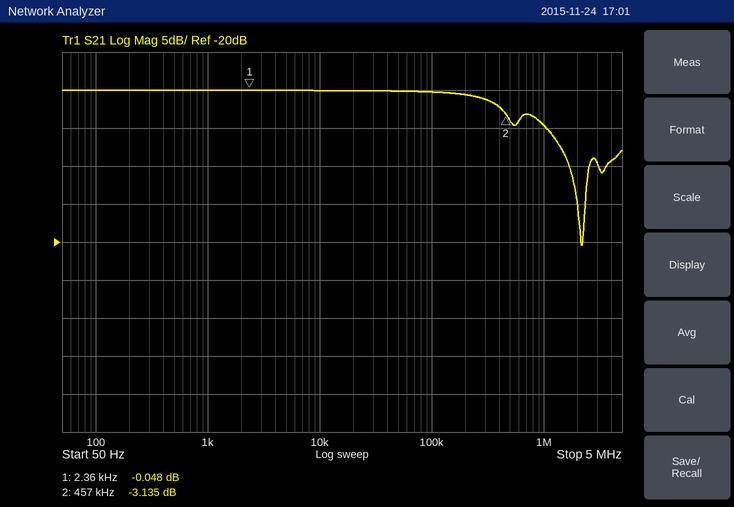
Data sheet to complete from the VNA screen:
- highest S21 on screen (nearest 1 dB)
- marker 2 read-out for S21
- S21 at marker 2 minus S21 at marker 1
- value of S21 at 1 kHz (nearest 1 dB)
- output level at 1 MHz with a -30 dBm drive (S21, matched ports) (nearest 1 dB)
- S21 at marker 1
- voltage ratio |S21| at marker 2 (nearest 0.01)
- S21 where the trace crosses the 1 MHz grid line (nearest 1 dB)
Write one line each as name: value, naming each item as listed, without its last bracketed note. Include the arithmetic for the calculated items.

highest S21 on screen: 0 dB
marker 2 read-out for S21: -3.135 dB
S21 at marker 2 minus S21 at marker 1: -3.135 − (-0.048) = -3.087 dB
value of S21 at 1 kHz: 0 dB
output level at 1 MHz with a -30 dBm drive (S21, matched ports): -30 dBm + (-5 dB) = -35 dBm
S21 at marker 1: -0.048 dB
voltage ratio |S21| at marker 2: 10^(-3.135/20) ≈ 0.70
S21 where the trace crosses the 1 MHz grid line: -5 dB
